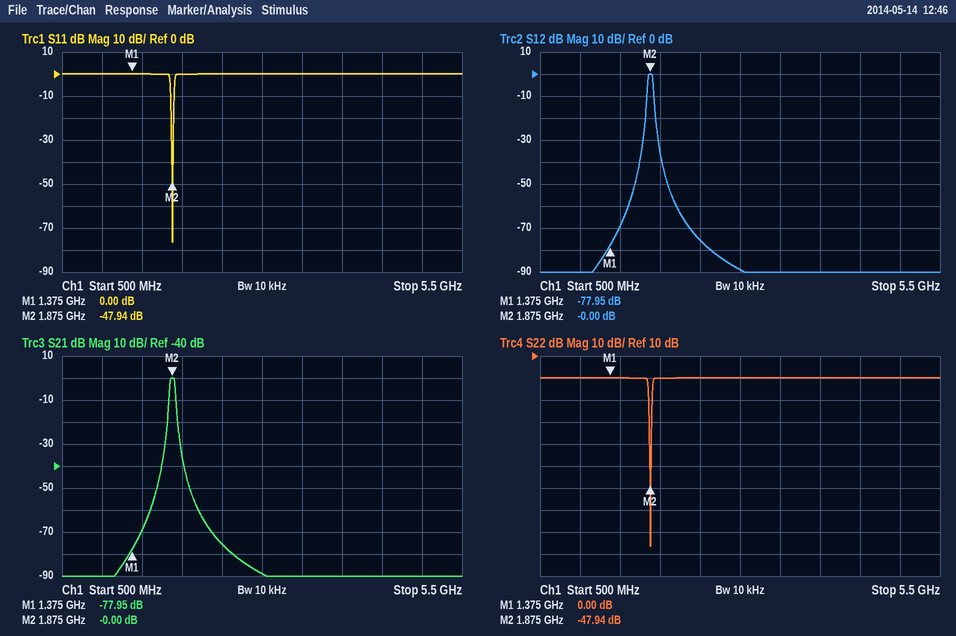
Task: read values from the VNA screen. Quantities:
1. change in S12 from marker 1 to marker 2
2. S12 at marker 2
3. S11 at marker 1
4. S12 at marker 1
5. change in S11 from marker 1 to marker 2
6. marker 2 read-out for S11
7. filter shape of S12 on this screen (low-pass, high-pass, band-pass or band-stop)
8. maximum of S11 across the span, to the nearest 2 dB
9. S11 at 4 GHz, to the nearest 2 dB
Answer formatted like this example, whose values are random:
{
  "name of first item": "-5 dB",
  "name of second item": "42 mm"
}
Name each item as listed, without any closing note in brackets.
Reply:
{
  "change in S12 from marker 1 to marker 2": "77.95 dB",
  "S12 at marker 2": "-0.00 dB",
  "S11 at marker 1": "0.00 dB",
  "S12 at marker 1": "-77.95 dB",
  "change in S11 from marker 1 to marker 2": "-47.94 dB",
  "marker 2 read-out for S11": "-47.94 dB",
  "filter shape of S12 on this screen": "band-pass",
  "maximum of S11 across the span, to the nearest 2 dB": "0 dB",
  "S11 at 4 GHz, to the nearest 2 dB": "0 dB"
}
